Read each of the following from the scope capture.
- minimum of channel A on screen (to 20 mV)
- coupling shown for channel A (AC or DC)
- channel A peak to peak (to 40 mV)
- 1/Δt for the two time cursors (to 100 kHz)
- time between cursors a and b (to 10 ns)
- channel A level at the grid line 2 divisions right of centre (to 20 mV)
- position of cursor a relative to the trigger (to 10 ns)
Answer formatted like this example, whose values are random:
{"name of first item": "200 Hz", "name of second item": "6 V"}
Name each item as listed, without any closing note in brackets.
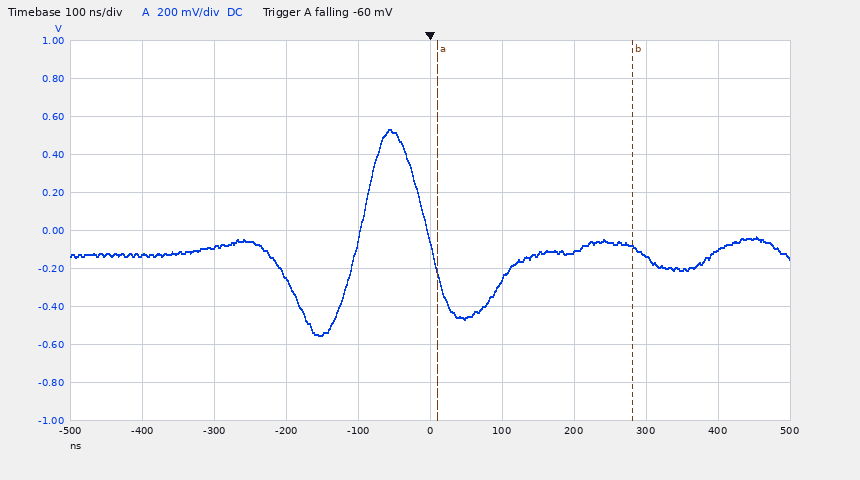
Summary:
{"minimum of channel A on screen": "-560 mV", "coupling shown for channel A": "DC", "channel A peak to peak": "1.08 V", "1/Δt for the two time cursors": "3.7 MHz", "time between cursors a and b": "270 ns", "channel A level at the grid line 2 divisions right of centre": "-120 mV", "position of cursor a relative to the trigger": "+10 ns"}
